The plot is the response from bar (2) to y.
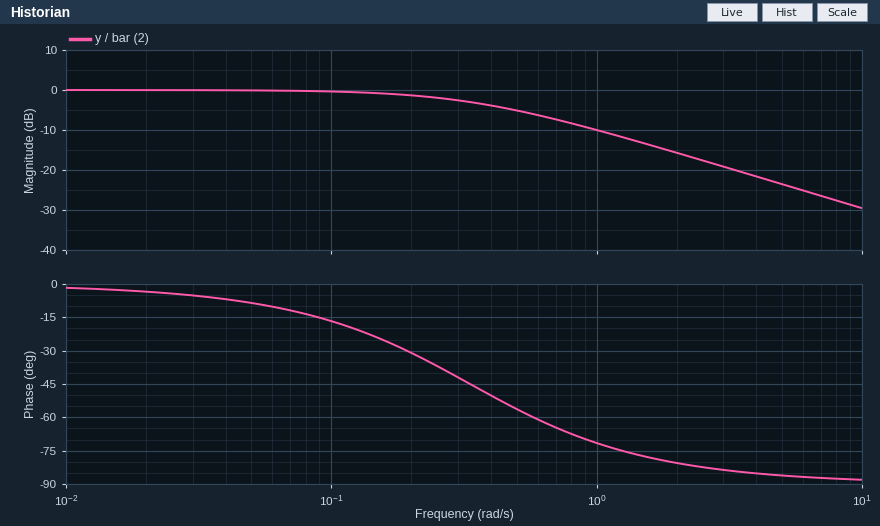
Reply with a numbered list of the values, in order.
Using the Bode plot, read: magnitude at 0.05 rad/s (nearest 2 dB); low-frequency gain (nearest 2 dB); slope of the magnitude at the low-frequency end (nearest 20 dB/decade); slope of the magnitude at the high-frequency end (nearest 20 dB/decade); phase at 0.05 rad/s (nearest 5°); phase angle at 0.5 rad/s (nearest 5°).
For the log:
1. 0 dB
2. 0 dB
3. 0 dB/decade
4. -20 dB/decade
5. -10°
6. -55°
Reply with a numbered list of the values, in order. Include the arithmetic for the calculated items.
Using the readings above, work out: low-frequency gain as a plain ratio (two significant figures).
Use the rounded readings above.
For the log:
1. 10^(0 / 20) = 1.0
